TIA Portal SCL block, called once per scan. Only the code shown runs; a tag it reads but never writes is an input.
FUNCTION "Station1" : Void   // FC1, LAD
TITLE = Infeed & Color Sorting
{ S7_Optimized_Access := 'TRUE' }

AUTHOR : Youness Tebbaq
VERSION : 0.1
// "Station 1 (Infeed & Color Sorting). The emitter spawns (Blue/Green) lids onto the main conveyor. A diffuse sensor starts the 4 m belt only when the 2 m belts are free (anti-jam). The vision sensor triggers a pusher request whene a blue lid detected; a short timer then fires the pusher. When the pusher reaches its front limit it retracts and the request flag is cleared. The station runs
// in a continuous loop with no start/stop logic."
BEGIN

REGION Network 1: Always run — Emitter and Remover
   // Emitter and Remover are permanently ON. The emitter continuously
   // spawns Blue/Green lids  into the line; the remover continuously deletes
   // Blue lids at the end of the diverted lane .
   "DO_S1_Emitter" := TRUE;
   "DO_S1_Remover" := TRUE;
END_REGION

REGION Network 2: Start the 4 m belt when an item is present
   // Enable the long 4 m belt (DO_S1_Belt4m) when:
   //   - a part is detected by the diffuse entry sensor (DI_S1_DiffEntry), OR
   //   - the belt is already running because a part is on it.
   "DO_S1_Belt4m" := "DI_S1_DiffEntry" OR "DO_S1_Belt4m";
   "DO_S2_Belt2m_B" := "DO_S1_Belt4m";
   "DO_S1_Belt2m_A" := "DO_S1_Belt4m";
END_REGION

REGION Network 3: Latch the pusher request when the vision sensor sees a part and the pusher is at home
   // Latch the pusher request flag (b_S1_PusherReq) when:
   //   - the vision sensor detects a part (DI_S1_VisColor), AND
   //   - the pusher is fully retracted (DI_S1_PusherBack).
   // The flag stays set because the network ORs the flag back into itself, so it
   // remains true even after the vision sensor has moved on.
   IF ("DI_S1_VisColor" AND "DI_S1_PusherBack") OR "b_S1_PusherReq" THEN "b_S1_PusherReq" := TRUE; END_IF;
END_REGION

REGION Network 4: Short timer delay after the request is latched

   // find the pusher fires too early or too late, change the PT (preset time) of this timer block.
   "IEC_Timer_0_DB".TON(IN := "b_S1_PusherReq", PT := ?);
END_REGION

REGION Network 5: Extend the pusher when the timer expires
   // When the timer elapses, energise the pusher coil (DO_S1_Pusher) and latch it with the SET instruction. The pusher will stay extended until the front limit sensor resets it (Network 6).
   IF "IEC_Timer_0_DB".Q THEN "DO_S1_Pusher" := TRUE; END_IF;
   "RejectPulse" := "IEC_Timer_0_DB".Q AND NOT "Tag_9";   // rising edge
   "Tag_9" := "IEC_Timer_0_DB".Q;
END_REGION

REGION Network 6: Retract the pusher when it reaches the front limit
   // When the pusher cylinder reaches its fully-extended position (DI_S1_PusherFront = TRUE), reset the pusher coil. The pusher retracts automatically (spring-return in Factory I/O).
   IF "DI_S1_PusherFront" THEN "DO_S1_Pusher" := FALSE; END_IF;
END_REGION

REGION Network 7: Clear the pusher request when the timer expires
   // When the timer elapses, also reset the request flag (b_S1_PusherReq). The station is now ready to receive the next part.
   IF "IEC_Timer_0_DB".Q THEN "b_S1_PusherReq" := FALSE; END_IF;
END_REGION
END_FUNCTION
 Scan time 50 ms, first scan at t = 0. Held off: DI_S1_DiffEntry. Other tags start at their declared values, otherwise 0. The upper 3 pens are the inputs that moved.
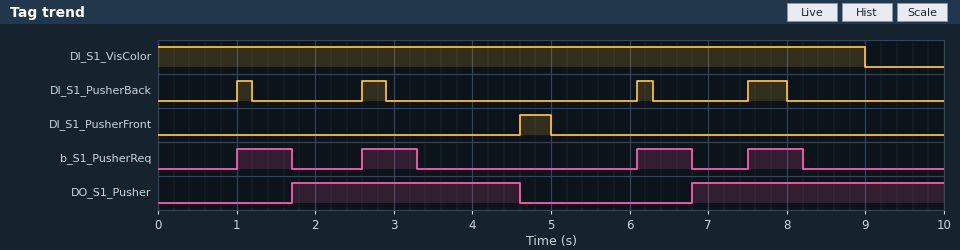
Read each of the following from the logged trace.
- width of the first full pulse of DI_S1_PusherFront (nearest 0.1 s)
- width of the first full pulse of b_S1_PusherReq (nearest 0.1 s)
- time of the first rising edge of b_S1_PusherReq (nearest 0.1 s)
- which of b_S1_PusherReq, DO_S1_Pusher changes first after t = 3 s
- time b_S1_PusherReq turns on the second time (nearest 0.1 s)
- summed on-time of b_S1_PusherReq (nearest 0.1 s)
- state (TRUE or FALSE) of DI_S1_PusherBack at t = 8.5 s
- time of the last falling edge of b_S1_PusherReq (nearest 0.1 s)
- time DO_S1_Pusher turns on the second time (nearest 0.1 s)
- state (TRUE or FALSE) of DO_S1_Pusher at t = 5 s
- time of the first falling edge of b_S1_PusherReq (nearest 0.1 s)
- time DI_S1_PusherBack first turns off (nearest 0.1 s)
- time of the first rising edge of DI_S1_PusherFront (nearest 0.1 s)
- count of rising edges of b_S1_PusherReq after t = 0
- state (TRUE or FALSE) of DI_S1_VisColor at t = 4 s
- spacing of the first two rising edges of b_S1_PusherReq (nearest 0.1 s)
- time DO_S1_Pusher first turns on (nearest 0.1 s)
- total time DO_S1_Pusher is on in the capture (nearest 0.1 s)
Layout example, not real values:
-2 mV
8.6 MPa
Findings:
0.4 s
0.7 s
1.0 s
b_S1_PusherReq
2.6 s
2.8 s
FALSE
8.2 s
6.8 s
FALSE
1.7 s
1.2 s
4.6 s
4
TRUE
1.6 s
1.7 s
6.1 s
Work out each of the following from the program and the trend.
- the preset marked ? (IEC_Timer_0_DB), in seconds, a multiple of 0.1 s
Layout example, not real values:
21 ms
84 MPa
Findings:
0.7 s
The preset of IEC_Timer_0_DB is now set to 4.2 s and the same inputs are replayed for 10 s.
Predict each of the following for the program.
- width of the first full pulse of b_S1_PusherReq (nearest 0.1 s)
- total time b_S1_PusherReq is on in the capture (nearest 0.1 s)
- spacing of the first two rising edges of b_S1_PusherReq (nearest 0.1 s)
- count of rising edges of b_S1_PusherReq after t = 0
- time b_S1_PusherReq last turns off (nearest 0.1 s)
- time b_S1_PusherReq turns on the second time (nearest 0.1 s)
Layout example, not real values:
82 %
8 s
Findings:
4.2 s
8.1 s
5.1 s
2
5.2 s
6.1 s
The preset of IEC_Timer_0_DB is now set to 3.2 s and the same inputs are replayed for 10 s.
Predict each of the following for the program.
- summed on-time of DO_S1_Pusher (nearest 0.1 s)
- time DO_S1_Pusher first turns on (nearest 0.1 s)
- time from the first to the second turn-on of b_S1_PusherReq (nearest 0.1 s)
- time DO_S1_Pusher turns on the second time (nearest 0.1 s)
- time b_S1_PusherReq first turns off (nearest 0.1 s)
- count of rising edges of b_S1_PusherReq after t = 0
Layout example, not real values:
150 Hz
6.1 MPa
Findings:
1.1 s
4.2 s
5.1 s
9.3 s
4.2 s
2
